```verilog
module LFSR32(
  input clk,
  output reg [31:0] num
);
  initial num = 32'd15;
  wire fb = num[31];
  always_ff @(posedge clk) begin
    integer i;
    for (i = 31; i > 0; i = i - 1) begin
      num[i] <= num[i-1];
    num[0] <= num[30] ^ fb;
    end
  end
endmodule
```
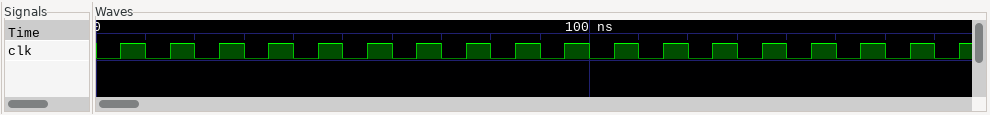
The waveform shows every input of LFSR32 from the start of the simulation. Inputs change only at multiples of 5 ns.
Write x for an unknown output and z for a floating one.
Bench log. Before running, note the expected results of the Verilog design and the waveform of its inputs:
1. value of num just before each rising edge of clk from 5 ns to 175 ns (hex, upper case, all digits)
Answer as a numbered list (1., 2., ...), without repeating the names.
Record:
1. 0000000F, 0000001E, 0000003C, 00000078, 000000F0, 000001E0, 000003C0, 00000780, 00000F00, 00001E00, 00003C00, 00007800, 0000F000, 0001E000, 0003C000, 00078000, 000F0000, 001E0000
